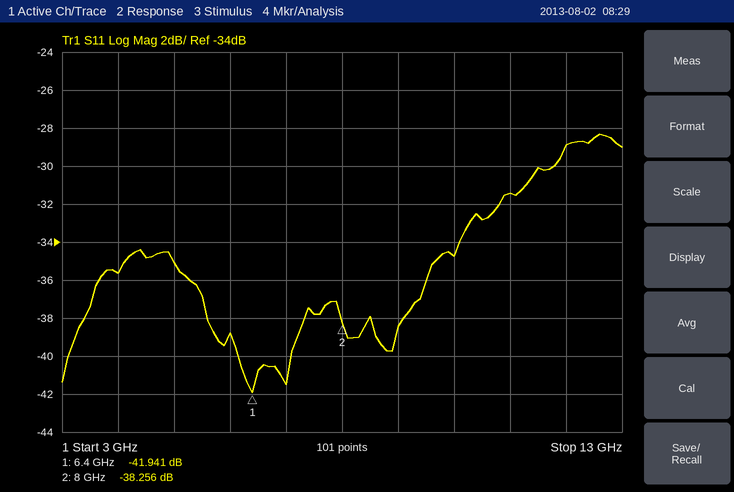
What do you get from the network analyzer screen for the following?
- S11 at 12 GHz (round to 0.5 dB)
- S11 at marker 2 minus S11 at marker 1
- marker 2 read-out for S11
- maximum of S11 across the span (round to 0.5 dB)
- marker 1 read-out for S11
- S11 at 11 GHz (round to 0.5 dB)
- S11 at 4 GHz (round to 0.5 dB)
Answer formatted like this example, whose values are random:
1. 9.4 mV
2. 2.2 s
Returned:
1. -29.0 dB
2. 3.685 dB
3. -38.256 dB
4. -28.5 dB
5. -41.941 dB
6. -31.5 dB
7. -35.5 dB
